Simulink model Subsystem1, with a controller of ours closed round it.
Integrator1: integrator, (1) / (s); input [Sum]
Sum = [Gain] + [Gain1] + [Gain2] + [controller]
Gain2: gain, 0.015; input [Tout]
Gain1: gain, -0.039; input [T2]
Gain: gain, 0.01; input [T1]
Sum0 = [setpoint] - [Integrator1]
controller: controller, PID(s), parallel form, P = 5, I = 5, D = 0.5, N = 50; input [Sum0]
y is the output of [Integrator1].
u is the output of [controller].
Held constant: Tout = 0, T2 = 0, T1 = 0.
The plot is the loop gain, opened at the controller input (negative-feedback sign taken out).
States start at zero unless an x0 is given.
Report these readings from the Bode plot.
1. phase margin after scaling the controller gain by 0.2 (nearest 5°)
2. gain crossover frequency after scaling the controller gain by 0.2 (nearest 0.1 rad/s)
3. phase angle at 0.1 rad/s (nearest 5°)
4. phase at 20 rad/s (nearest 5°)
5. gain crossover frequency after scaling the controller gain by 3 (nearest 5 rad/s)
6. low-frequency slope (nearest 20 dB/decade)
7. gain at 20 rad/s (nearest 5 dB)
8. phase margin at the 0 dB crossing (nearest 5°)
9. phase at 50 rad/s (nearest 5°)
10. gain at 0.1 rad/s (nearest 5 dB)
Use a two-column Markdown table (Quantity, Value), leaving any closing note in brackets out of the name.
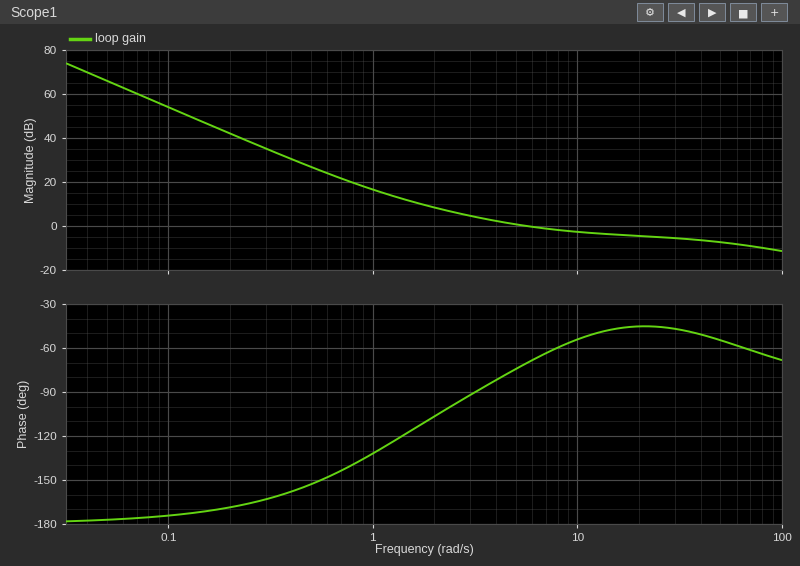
| Quantity | Value |
|---|---|
| phase margin after scaling the controller gain by 0.2 | 55° |
| gain crossover frequency after scaling the controller gain by 0.2 | 1.2 rad/s |
| phase angle at 0.1 rad/s | -175° |
| phase at 20 rad/s | -45° |
| gain crossover frequency after scaling the controller gain by 3 | 75 rad/s |
| low-frequency slope | -40 dB/decade |
| gain at 20 rad/s | -5 dB |
| phase margin at the 0 dB crossing | 110° |
| phase at 50 rad/s | -55° |
| gain at 0.1 rad/s | 55 dB |
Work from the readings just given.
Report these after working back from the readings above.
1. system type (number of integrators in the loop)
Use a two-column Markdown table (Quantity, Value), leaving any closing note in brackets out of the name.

| Quantity | Value |
|---|---|
| system type | 2 |
